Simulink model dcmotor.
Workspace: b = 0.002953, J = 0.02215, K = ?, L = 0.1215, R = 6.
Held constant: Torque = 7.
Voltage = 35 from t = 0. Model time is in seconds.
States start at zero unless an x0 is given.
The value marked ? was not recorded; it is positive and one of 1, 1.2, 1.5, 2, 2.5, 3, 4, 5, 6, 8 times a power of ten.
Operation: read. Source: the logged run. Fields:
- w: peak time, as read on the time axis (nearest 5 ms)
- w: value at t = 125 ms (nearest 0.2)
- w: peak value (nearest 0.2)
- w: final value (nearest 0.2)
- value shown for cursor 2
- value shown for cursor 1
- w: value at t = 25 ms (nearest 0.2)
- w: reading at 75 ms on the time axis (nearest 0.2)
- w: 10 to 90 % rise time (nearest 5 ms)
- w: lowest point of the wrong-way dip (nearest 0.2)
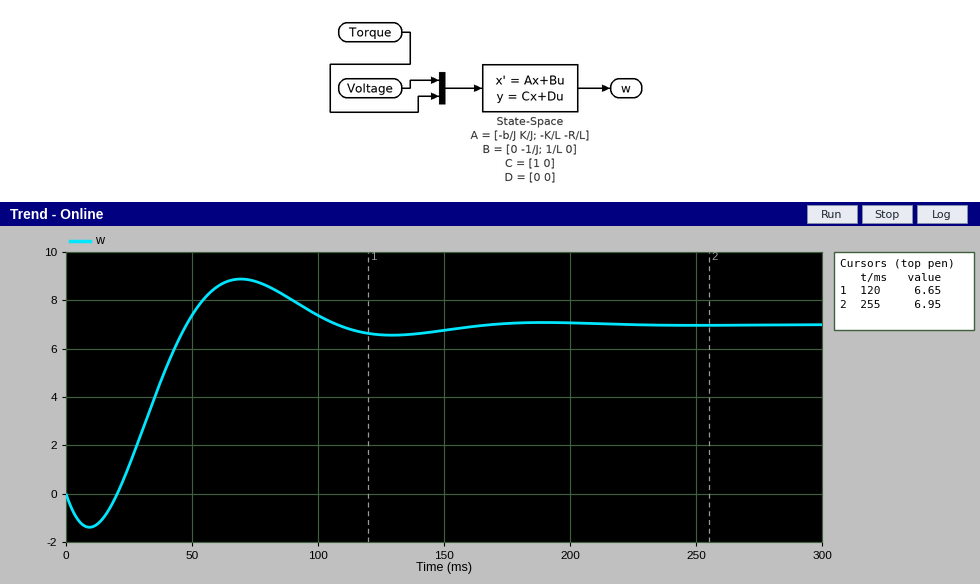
70 ms
6.6
8.8
7.0
6.95
6.65
1.2
8.8
20 ms
-1.4
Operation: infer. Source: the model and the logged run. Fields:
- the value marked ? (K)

3
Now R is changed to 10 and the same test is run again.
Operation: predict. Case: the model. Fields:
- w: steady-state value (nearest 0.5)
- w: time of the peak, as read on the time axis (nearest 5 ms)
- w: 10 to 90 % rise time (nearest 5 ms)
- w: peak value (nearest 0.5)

4.0
90 ms
30 ms
4.0
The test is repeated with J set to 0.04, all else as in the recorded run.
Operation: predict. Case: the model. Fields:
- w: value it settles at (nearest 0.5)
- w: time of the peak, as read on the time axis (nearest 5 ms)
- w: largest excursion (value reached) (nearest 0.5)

7.0
100 ms
8.0
